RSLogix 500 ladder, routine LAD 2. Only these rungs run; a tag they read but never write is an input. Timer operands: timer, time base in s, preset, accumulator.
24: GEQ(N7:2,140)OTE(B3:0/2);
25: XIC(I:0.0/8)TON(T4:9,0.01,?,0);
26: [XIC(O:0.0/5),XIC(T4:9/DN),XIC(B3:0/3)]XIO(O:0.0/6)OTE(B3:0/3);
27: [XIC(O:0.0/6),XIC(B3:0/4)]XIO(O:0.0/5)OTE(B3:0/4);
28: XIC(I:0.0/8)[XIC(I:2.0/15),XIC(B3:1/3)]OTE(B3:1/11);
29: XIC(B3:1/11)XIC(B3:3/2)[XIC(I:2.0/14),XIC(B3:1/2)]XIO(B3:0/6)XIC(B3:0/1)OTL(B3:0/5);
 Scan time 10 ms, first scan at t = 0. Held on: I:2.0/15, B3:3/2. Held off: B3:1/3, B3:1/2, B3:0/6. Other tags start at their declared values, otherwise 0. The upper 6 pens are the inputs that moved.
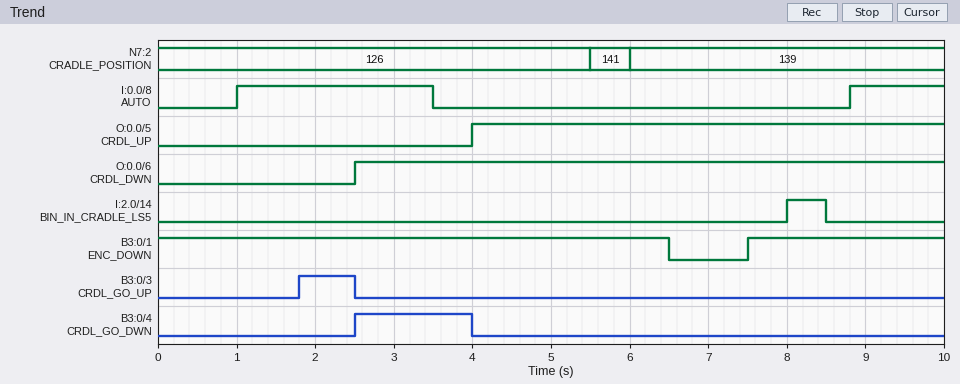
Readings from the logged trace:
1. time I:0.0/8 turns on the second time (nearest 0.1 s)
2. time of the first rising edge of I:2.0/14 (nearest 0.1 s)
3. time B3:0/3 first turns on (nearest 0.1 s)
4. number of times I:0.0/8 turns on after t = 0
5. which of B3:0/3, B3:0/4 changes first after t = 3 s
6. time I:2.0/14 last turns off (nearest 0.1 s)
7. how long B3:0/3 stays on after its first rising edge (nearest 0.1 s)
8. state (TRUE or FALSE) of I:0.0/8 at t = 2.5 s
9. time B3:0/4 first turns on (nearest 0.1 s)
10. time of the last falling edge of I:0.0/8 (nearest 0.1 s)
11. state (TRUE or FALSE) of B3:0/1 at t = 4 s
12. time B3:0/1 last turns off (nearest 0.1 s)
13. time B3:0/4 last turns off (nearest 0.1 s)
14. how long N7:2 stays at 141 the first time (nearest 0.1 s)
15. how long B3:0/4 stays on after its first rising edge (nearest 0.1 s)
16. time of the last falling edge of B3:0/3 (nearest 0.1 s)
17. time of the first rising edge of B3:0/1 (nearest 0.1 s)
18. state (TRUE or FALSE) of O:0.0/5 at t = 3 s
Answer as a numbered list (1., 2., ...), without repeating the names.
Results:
1. 8.8 s
2. 8.0 s
3. 1.8 s
4. 2
5. B3:0/4
6. 8.5 s
7. 0.7 s
8. TRUE
9. 2.5 s
10. 3.5 s
11. TRUE
12. 6.5 s
13. 4.0 s
14. 0.5 s
15. 1.5 s
16. 2.5 s
17. 7.5 s
18. FALSE
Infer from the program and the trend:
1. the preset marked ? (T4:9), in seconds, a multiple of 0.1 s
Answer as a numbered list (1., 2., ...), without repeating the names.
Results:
1. 0.8 s
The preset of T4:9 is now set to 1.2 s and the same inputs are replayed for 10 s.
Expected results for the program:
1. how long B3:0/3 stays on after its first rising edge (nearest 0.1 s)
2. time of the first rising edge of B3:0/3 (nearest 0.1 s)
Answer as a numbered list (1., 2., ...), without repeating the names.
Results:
1. 0.3 s
2. 2.2 s
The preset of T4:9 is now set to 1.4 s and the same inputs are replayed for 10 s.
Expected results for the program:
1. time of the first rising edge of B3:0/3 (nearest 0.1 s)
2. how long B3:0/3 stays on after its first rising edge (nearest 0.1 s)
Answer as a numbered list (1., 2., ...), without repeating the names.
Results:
1. 2.4 s
2. 0.1 s
